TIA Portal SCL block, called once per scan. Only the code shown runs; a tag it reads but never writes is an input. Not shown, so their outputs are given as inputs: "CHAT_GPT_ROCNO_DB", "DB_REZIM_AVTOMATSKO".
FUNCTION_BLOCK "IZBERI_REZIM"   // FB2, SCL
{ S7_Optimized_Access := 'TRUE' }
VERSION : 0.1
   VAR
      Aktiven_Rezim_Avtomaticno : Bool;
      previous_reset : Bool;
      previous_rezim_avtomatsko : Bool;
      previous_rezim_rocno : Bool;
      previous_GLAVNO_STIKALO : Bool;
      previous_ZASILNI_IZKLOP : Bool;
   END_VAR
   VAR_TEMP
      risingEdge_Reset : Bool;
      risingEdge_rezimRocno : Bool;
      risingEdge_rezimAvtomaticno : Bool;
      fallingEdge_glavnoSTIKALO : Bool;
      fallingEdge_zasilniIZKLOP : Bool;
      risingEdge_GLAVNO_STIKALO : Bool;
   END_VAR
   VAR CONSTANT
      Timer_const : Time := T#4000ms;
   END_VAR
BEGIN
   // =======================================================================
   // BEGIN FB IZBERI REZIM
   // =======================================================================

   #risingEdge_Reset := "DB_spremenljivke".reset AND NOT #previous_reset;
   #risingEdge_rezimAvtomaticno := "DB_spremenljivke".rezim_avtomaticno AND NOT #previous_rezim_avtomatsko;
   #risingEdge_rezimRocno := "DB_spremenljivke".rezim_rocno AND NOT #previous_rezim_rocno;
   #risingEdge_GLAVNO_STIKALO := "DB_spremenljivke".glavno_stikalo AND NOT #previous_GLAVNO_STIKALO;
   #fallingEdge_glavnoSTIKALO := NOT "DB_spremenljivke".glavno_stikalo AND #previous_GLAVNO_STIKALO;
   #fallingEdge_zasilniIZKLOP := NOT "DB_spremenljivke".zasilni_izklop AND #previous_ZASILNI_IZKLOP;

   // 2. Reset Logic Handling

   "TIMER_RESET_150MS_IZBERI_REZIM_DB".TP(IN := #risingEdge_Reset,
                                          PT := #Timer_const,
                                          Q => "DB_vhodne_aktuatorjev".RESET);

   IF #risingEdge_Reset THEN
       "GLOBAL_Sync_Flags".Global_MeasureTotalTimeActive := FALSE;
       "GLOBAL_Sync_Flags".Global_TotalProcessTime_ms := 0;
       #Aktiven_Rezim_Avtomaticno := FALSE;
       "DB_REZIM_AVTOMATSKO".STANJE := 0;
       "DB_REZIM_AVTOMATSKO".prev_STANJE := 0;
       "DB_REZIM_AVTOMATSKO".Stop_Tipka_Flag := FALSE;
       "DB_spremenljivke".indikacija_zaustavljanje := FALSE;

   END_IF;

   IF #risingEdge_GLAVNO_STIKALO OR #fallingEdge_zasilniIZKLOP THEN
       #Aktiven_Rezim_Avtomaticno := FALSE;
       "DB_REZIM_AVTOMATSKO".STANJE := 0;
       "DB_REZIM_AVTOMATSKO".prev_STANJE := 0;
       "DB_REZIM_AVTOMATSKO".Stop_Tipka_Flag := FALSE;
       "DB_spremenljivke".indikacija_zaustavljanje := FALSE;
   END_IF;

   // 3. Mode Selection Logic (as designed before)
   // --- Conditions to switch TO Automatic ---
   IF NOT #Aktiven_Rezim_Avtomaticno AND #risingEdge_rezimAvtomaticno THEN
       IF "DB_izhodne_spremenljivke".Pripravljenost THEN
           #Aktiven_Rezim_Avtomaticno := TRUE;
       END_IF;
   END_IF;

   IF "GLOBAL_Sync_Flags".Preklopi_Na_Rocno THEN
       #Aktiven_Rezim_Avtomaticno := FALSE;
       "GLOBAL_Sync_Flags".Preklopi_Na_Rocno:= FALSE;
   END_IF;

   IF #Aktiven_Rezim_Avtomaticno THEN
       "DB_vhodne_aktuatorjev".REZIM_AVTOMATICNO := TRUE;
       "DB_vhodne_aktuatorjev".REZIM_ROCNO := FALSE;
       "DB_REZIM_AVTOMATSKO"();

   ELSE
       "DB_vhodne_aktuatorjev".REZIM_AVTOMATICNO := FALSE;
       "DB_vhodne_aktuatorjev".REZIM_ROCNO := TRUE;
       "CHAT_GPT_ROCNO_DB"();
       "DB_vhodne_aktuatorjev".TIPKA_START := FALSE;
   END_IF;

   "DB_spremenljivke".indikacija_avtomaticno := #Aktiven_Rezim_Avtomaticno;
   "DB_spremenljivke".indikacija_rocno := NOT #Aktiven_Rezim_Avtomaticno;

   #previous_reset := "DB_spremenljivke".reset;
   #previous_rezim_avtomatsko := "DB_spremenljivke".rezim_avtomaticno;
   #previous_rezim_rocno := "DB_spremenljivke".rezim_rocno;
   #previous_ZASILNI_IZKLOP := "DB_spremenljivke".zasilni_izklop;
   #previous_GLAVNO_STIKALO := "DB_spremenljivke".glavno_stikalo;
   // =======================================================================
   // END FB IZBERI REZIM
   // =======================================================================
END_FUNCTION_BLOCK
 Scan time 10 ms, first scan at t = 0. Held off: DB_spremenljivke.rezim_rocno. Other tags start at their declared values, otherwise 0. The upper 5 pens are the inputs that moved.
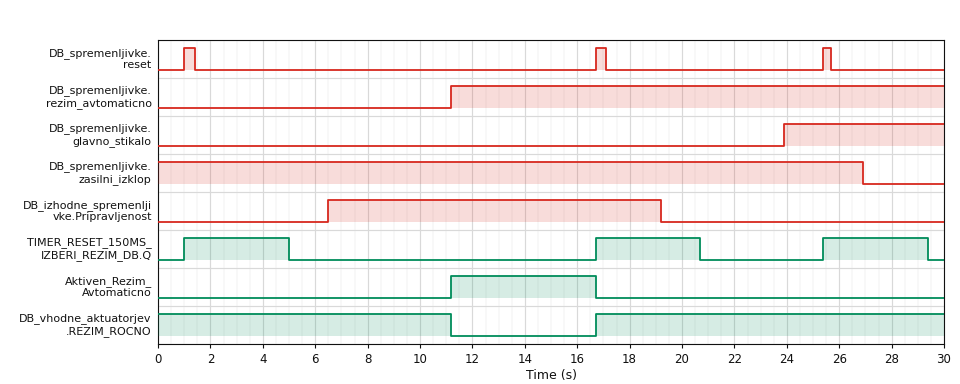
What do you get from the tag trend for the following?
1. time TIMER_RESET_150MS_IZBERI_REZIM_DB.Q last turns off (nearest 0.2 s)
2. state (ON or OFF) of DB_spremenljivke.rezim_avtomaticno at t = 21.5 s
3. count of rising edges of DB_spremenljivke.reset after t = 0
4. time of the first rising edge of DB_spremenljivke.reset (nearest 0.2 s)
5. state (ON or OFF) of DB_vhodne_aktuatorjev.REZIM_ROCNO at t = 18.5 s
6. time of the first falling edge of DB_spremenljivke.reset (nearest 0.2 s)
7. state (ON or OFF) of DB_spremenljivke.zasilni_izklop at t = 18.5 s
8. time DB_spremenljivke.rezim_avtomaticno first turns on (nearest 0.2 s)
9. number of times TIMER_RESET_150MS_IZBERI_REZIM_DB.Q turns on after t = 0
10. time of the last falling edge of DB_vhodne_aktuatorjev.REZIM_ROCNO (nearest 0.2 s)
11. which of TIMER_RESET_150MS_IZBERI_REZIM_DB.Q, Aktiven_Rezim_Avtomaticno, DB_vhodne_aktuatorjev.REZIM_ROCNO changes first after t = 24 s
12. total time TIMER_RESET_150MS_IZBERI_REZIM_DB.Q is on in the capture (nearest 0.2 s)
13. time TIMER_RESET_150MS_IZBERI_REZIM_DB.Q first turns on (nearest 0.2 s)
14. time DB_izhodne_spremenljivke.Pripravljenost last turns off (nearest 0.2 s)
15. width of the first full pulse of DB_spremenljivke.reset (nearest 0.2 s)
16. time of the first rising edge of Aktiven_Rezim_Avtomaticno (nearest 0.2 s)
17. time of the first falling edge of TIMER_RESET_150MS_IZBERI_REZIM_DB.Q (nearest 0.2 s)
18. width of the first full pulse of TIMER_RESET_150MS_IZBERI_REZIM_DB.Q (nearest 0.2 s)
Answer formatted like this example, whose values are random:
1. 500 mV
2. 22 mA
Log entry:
1. 29.4 s
2. ON
3. 3
4. 1.0 s
5. ON
6. 1.4 s
7. ON
8. 11.2 s
9. 3
10. 11.2 s
11. TIMER_RESET_150MS_IZBERI_REZIM_DB.Q
12. 12.0 s
13. 1.0 s
14. 19.2 s
15. 0.4 s
16. 11.2 s
17. 5.0 s
18. 4.0 s
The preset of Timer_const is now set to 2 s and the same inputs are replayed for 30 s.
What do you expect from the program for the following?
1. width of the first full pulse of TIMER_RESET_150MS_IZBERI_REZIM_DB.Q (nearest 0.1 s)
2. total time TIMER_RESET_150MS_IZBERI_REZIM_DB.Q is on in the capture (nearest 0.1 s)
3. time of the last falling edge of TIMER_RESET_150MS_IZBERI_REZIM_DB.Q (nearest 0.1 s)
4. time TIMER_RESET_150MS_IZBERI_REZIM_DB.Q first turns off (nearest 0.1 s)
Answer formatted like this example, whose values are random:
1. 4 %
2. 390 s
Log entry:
1. 2.0 s
2. 6.0 s
3. 27.4 s
4. 3.0 s
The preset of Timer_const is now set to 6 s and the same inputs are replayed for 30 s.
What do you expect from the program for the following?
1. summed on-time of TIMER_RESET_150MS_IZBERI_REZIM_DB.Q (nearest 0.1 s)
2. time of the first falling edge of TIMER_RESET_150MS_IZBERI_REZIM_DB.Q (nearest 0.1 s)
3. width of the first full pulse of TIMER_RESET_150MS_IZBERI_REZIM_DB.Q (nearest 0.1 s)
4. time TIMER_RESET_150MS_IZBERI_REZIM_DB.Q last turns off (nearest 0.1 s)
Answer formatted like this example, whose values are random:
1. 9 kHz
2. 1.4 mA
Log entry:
1. 16.6 s
2. 7.0 s
3. 6.0 s
4. 22.7 s
